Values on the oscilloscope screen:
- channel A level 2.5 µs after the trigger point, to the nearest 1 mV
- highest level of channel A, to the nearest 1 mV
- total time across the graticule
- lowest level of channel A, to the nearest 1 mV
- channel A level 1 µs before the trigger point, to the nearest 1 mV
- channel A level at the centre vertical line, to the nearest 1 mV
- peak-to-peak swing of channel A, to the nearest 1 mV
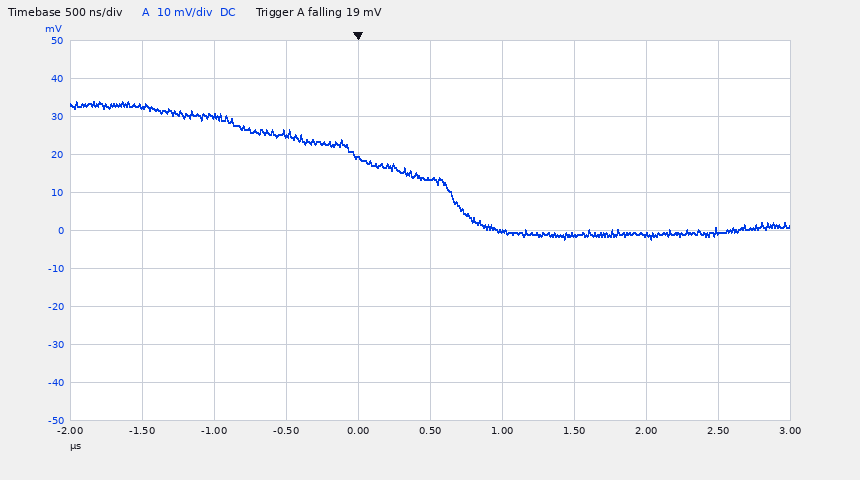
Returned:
0 mV
34 mV
5 µs
-2 mV
30 mV
14 mV
36 mV
